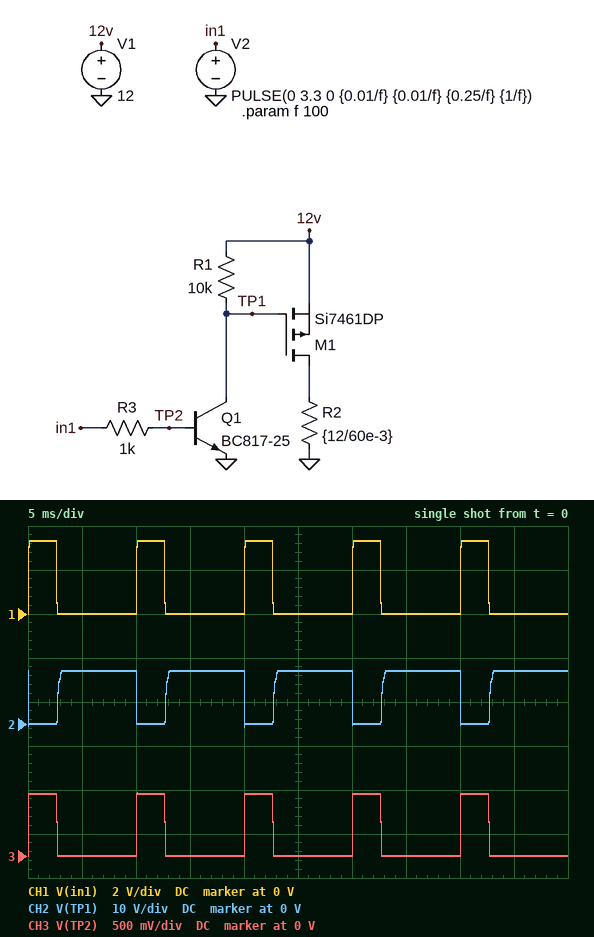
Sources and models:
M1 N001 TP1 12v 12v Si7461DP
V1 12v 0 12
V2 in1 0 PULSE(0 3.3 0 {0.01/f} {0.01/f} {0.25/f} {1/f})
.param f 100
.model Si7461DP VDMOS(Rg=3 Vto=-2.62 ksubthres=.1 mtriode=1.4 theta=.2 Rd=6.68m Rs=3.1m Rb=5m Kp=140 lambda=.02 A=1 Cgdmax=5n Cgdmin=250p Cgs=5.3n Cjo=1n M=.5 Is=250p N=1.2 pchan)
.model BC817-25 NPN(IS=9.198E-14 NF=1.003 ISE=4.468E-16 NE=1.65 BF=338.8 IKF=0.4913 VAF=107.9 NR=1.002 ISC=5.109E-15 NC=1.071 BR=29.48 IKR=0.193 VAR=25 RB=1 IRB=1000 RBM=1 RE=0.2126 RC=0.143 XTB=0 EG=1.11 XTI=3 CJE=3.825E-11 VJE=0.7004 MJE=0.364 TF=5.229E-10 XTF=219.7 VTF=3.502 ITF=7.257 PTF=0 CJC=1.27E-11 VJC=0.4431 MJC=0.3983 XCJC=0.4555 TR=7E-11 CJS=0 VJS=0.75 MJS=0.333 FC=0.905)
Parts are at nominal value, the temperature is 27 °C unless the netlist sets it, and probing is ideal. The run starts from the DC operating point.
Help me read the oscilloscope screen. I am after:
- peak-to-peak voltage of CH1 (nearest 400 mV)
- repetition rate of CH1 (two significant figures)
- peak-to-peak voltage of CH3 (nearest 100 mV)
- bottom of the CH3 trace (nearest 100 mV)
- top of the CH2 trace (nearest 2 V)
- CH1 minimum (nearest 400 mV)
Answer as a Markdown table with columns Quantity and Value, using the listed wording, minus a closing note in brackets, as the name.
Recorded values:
| Quantity | Value |
|---|---|
| peak-to-peak voltage of CH1 | 3.2 V |
| repetition rate of CH1 | 100 Hz |
| peak-to-peak voltage of CH3 | 700 mV |
| bottom of the CH3 trace | 0 V |
| top of the CH2 trace | 12 V |
| CH1 minimum | 0 V |
